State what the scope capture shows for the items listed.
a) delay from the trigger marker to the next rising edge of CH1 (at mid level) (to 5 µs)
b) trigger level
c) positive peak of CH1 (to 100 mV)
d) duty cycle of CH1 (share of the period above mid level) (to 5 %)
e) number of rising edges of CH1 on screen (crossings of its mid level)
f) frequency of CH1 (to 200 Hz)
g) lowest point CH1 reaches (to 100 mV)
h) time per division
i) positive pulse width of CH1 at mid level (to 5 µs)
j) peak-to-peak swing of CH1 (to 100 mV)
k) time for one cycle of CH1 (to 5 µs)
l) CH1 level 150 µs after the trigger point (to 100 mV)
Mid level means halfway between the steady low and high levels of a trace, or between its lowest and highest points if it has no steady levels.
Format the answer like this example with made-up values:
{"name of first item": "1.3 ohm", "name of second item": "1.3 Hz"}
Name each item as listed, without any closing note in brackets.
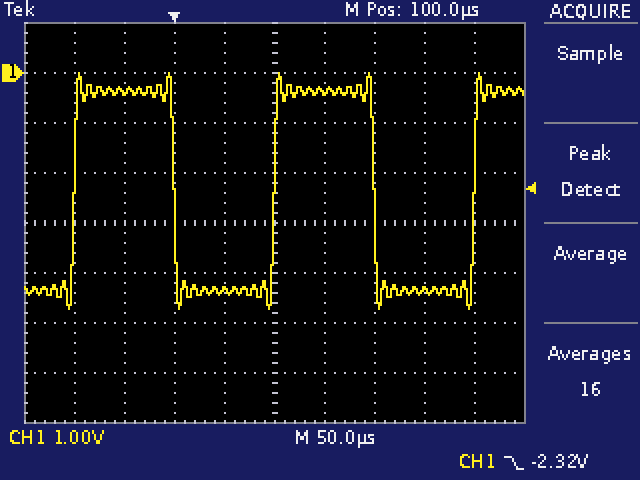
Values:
{"delay from the trigger marker to the next rising edge of CH1 (at mid level)": "100 µs", "trigger level": "-2.32 V", "positive peak of CH1": "0.0 V", "duty cycle of CH1 (share of the period above mid level)": "50 %", "number of rising edges of CH1 on screen": "3", "frequency of CH1": "5.0 kHz", "lowest point CH1 reaches": "-4.7 V", "time per division": "50 µs", "positive pulse width of CH1 at mid level": "100 µs", "peak-to-peak swing of CH1": "4.7 V", "time for one cycle of CH1": "200 µs", "CH1 level 150 µs after the trigger point": "-400 mV"}
